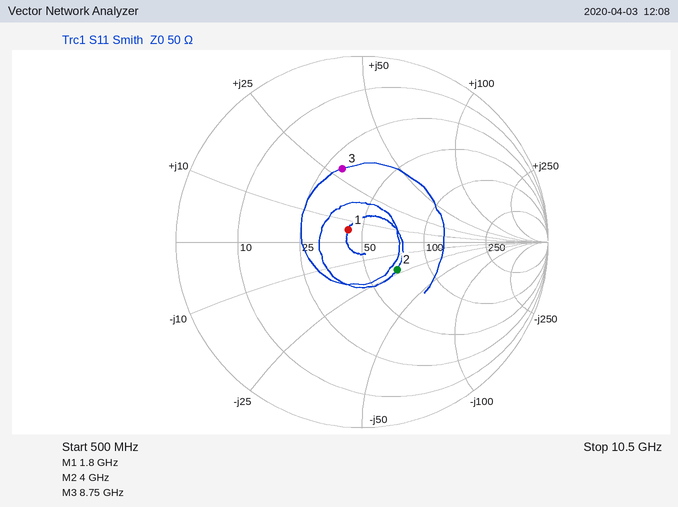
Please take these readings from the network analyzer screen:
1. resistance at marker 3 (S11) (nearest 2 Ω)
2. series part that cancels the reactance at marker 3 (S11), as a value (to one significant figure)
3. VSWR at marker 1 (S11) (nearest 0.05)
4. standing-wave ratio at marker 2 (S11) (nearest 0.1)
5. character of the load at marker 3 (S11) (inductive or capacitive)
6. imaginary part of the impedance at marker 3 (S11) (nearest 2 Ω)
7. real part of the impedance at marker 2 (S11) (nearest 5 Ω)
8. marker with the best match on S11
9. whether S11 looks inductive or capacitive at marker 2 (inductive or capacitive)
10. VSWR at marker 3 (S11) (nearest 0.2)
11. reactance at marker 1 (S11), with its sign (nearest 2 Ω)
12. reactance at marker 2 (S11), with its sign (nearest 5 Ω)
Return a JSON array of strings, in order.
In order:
["30 Ω", "600 fF", "1.20", "1.6", "inductive", "+28 Ω", "70 Ω", "marker 1", "capacitive", "2.4", "+6 Ω", "-20 Ω"]
